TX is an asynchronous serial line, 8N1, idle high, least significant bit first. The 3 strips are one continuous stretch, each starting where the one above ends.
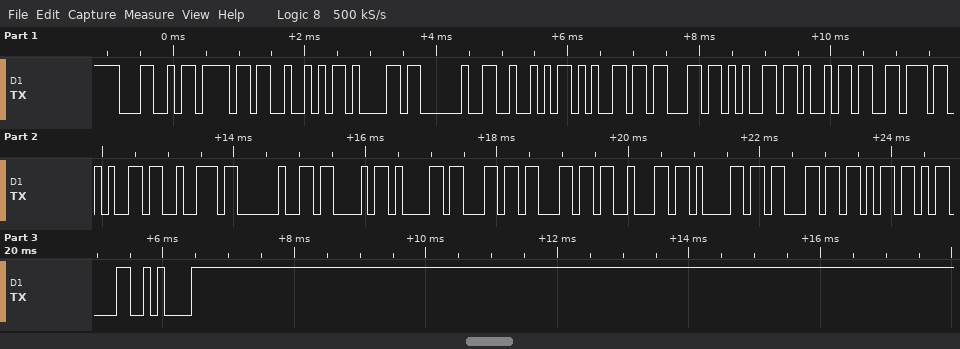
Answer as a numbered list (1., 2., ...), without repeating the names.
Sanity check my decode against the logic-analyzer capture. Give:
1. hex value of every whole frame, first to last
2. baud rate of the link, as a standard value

1. 0x4C 0x6F 0x52 0x61 0x20 0x52 0x65 0x63 0x65 0x69 0x76 0x65 0x72 0x20 0x43 0x61 0x6C 0x6C 0x62 0x61 0x63 0x6B 0x0D 0x0A
2. 9600 baud
